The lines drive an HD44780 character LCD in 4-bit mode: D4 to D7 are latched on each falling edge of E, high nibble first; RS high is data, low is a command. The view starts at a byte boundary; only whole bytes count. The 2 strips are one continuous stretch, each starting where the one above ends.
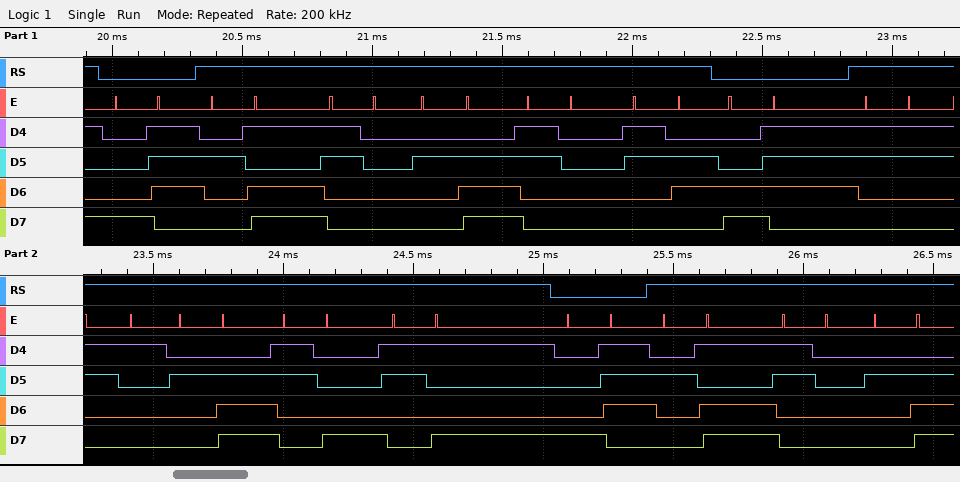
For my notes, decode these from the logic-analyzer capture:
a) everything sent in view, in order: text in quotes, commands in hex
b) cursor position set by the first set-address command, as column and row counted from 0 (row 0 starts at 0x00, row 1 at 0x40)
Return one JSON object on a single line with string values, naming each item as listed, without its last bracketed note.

{"everything sent in view, in order: text in quotes, commands in hex": "0x87 \"-0.06\" 0xC7 \"31.89\" 0x87 \"-0.\"", "cursor position set by the first set-address command, as column and row counted from 0": "column 7, row 0"}
